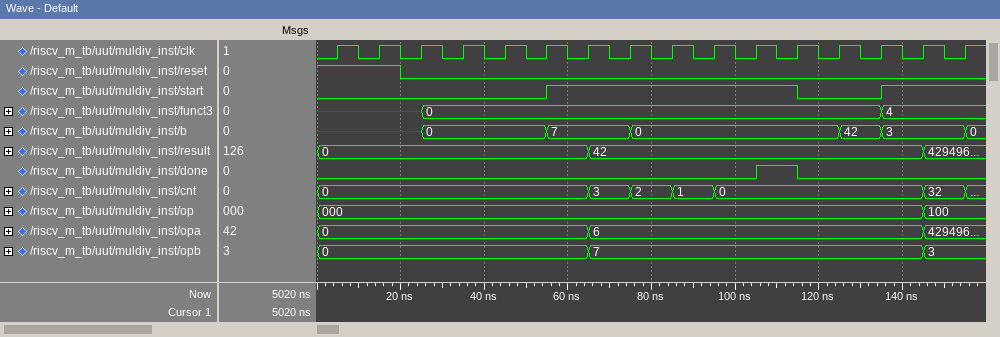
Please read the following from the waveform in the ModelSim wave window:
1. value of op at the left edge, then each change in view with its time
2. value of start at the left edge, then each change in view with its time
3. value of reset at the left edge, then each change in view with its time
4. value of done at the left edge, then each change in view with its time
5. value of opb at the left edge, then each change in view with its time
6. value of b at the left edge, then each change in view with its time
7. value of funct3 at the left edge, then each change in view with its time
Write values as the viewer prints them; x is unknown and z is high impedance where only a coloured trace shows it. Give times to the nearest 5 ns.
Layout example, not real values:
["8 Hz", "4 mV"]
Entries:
["000, 100 at 145 ns", "0, 1 at 55 ns, 0 at 115 ns, 1 at 135 ns", "1, 0 at 20 ns", "0, 1 at 105 ns, 0 at 115 ns", "0, 7 at 65 ns, 3 at 145 ns", "x, 0 at 25 ns, 7 at 55 ns, 0 at 75 ns, 42 at 125 ns, 3 at 135 ns, 0 at 155 ns", "x, 0 at 25 ns, 4 at 135 ns"]
